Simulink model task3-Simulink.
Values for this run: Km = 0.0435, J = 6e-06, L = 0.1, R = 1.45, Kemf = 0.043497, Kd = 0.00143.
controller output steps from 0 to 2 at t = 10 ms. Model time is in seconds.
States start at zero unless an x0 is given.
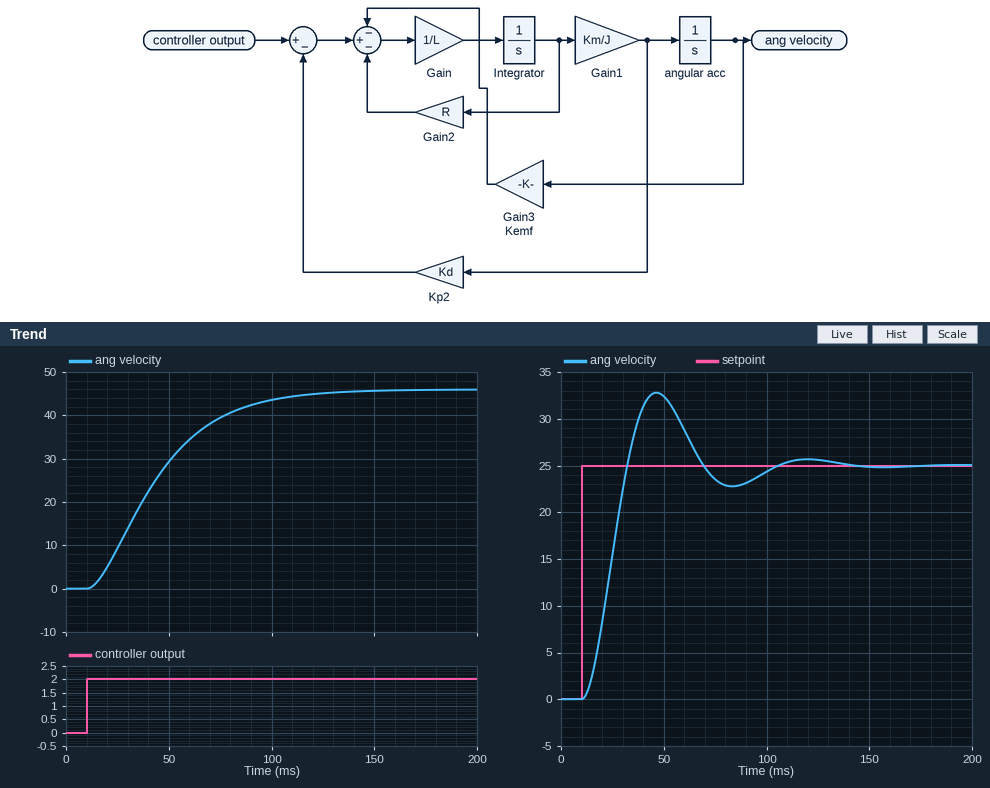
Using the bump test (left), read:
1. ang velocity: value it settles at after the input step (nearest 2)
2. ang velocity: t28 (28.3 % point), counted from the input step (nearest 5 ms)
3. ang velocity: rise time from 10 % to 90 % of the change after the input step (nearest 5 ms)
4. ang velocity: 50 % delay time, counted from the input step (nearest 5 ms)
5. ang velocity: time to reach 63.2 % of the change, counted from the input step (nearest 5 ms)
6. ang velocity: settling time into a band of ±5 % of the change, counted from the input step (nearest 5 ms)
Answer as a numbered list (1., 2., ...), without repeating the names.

1. 46
2. 20 ms
3. 65 ms
4. 30 ms
5. 40 ms
6. 90 ms
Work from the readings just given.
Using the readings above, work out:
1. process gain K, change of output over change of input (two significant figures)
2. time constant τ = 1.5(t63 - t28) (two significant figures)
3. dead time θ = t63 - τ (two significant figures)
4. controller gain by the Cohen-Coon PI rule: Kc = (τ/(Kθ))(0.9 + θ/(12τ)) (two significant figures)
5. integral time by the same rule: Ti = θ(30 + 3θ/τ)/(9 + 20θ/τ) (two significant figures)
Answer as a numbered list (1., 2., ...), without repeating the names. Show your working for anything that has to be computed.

1. (46 - 0) / 2 = 23
2. 1.5 × (40 - 20) = 30 ms
3. 40 - 30 = 10 ms
4. 30 / (23 × 10) × (0.9 + 10 / (12 × 30)) = 0.12
5. 10 × (30 + 3 × 10 / 30) / (9 + 20 × 10 / 30) = 20 ms
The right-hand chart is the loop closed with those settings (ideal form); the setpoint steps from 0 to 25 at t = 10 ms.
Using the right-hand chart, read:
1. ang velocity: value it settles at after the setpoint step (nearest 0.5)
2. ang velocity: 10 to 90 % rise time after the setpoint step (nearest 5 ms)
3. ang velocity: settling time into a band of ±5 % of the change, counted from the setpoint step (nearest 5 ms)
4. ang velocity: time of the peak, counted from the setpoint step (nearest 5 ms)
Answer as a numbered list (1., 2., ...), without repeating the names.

1. 25.0
2. 15 ms
3. 85 ms
4. 35 ms
